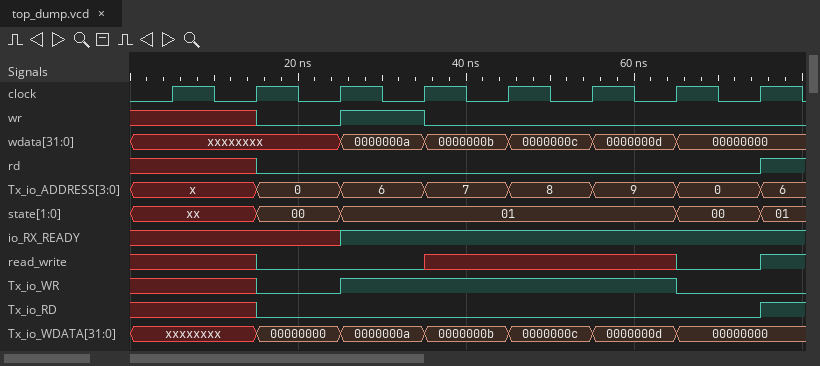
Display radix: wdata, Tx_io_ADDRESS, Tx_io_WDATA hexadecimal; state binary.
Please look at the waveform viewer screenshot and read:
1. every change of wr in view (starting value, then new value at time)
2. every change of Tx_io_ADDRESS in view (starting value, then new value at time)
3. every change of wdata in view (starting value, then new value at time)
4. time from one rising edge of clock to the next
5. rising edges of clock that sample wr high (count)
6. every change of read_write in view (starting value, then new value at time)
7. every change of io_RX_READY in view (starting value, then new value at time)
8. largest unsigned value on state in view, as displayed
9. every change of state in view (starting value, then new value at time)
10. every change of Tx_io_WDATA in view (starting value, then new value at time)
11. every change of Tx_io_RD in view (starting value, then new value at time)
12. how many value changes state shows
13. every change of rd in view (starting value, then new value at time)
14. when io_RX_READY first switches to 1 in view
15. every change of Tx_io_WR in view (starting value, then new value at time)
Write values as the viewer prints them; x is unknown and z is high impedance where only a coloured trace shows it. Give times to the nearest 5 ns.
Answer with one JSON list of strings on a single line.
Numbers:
["x, 0 at 15 ns, 1 at 25 ns, 0 at 35 ns", "x, 0 at 15 ns, 6 at 25 ns, 7 at 35 ns, 8 at 45 ns, 9 at 55 ns, 0 at 65 ns, 6 at 75 ns", "xxxxxxxx, 0000000a at 25 ns, 0000000b at 35 ns, 0000000c at 45 ns, 0000000d at 55 ns, 00000000 at 65 ns", "10 ns", "1", "x, 0 at 15 ns, x at 35 ns, 0 at 65 ns, 1 at 75 ns", "x, 1 at 25 ns", "01", "xx, 00 at 15 ns, 01 at 25 ns, 00 at 65 ns, 01 at 75 ns", "xxxxxxxx, 00000000 at 15 ns, 0000000a at 25 ns, 0000000b at 35 ns, 0000000c at 45 ns, 0000000d at 55 ns, 00000000 at 65 ns", "x, 0 at 15 ns, 1 at 75 ns", "4", "x, 0 at 15 ns, 1 at 75 ns", "25 ns", "x, 0 at 15 ns, 1 at 25 ns, 0 at 65 ns"]
